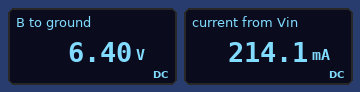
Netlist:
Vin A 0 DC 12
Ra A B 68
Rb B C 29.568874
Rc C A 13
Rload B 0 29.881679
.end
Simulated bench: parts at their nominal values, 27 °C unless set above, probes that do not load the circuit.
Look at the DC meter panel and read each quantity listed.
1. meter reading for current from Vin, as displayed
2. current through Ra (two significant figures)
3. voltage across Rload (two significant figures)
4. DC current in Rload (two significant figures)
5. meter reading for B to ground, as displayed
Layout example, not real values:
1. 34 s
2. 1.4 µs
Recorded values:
1. 214.1 mA
2. 82 mA
3. 6.4 V
4. 210 mA
5. 6.40 V
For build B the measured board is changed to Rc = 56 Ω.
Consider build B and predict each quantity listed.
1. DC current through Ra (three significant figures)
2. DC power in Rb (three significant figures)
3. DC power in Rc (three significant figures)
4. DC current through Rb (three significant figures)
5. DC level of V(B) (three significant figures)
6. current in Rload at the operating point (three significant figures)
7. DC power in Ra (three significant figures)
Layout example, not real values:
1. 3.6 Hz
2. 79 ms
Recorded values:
1. 98.7 mA
2. 182 mW
3. 344 mW
4. 78.4 mA
5. 5.29 V
6. 177 mA
7. 662 mW
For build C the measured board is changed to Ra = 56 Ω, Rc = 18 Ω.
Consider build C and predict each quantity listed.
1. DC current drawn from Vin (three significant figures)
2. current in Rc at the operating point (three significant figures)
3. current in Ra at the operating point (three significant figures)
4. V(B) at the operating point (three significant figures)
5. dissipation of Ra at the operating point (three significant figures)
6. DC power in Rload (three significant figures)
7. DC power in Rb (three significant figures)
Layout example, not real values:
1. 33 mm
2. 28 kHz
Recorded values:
1. 216 mA
2. 117 mA
3. 99.1 mA
4. 6.45 V
5. 550 mW
6. 1.39 W
7. 403 mW
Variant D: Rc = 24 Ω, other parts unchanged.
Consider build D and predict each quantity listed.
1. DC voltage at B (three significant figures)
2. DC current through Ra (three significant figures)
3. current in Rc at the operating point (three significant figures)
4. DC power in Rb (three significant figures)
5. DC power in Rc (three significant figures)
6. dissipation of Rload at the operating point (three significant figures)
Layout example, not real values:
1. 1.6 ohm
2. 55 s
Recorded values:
1. 5.99 V
2. 88.4 mA
3. 112 mA
4. 372 mW
5. 302 mW
6. 1.20 W
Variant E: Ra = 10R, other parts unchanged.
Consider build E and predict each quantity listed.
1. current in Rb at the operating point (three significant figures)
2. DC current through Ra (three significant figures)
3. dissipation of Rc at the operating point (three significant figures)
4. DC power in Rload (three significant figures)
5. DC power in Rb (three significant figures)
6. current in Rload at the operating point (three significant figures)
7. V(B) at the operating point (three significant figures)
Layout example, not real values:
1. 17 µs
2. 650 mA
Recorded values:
1. 60.1 mA
2. 256 mA
3. 47.0 mW
4. 2.98 W
5. 107 mW
6. 316 mA
7. 9.44 V
